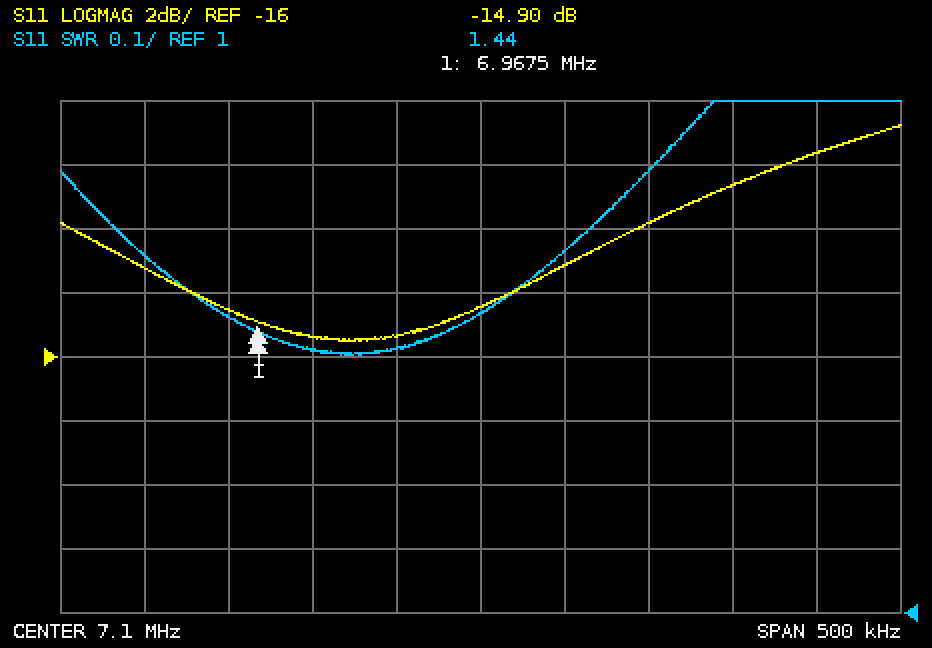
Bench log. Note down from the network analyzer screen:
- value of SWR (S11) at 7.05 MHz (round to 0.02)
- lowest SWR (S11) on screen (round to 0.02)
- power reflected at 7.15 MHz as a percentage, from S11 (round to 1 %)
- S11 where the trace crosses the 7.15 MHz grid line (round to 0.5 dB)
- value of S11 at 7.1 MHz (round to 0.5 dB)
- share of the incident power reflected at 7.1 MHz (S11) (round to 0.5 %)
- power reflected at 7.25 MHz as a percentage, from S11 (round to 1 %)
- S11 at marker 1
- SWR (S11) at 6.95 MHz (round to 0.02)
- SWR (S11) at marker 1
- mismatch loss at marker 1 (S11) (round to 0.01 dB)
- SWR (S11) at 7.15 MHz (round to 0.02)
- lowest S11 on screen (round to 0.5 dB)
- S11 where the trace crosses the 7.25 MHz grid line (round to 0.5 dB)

1.42
1.40
5 %
-13.0 dB
-14.5 dB
3.5 %
9 %
-14.90 dB
1.46
1.44
0.14 dB
1.56
-15.5 dB
-10.5 dB
